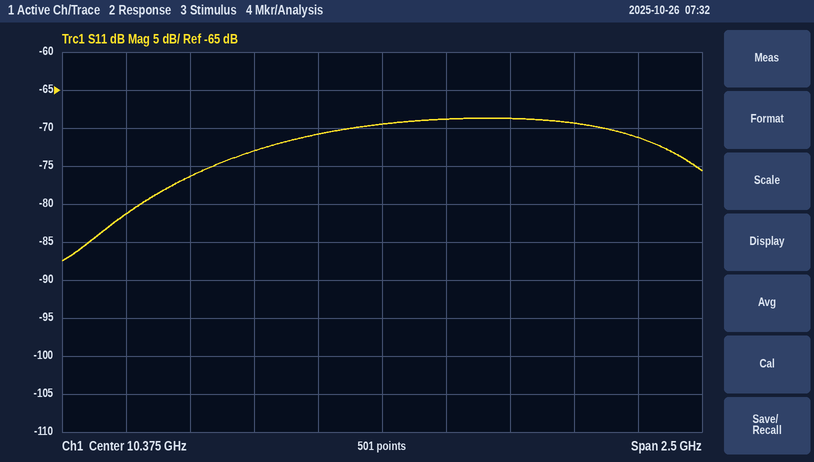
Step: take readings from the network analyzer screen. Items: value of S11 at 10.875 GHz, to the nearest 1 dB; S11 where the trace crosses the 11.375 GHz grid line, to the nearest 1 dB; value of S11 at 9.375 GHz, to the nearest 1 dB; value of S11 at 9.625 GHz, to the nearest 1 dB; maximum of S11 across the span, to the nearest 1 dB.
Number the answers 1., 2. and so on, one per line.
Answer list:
1. -69 dB
2. -71 dB
3. -81 dB
4. -76 dB
5. -69 dB
